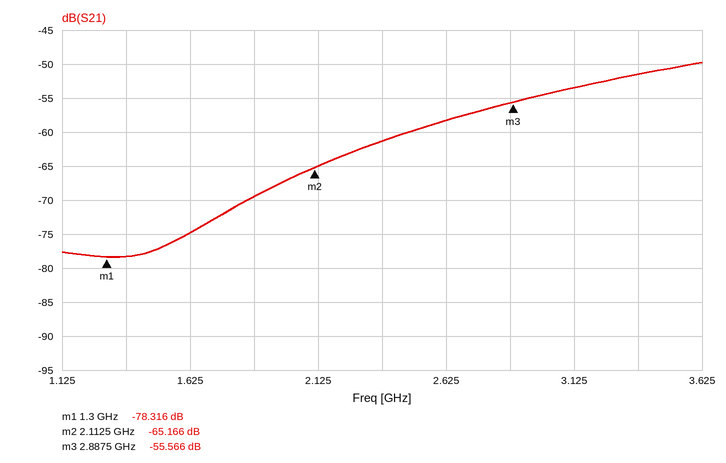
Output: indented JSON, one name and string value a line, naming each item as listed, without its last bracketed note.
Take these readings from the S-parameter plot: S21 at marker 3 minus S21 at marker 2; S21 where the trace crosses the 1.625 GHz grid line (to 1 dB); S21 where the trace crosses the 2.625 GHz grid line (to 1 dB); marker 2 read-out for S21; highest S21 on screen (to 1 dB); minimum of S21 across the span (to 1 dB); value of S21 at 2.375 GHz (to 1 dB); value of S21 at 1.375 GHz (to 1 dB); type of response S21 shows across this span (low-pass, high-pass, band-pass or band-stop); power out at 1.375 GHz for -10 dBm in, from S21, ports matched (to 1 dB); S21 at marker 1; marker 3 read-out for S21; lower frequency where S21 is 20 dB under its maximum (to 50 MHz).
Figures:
{
  "S21 at marker 3 minus S21 at marker 2": "9.600 dB",
  "S21 where the trace crosses the 1.625 GHz grid line": "-75 dB",
  "S21 where the trace crosses the 2.625 GHz grid line": "-58 dB",
  "marker 2 read-out for S21": "-65.166 dB",
  "highest S21 on screen": "-50 dB",
  "minimum of S21 across the span": "-78 dB",
  "value of S21 at 2.375 GHz": "-61 dB",
  "value of S21 at 1.375 GHz": "-78 dB",
  "type of response S21 shows across this span": "high-pass",
  "power out at 1.375 GHz for -10 dBm in, from S21, ports matched": "-88 dBm",
  "S21 at marker 1": "-78.316 dB",
  "marker 3 read-out for S21": "-55.566 dB",
  "lower frequency where S21 is 20 dB under its maximum": "1.85 GHz"
}
